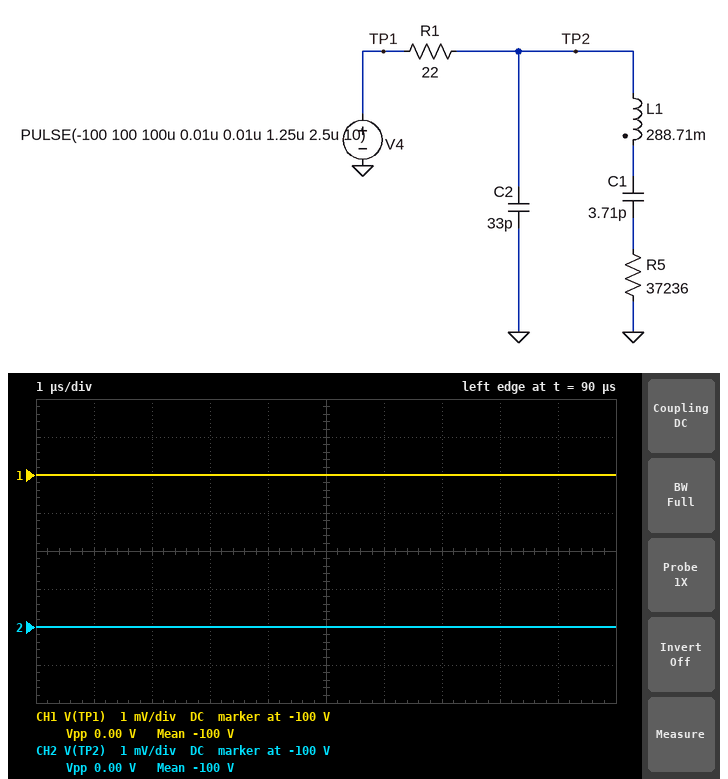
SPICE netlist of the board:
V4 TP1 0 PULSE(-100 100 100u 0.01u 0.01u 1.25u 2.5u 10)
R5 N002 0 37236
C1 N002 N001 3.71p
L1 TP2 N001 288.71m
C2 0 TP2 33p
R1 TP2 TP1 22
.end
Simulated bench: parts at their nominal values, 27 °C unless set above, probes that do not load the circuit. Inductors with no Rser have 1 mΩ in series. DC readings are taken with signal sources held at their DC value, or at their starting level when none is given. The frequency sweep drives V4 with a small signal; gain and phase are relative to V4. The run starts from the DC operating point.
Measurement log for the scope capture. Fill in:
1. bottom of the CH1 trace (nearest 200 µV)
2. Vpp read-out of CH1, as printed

-100.0000 V
0.00 V
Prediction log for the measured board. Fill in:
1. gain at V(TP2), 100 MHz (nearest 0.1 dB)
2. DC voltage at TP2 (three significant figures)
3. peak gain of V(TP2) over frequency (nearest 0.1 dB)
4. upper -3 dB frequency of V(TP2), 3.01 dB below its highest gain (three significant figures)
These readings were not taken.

-0.8 dB
-100 V
0 dB
219 MHz
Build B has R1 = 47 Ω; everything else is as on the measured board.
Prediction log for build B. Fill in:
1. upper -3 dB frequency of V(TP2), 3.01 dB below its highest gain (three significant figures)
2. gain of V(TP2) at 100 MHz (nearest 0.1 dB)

103 MHz
-2.9 dB
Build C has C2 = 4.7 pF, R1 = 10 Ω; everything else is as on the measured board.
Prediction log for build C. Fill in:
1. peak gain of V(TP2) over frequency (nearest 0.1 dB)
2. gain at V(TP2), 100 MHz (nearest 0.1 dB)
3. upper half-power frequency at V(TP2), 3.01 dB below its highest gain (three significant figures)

0 dB
0 dB
3.39 GHz
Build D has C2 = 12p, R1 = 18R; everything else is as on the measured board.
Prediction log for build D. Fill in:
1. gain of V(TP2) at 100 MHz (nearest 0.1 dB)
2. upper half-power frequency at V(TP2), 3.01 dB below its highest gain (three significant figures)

-0.1 dB
737 MHz
